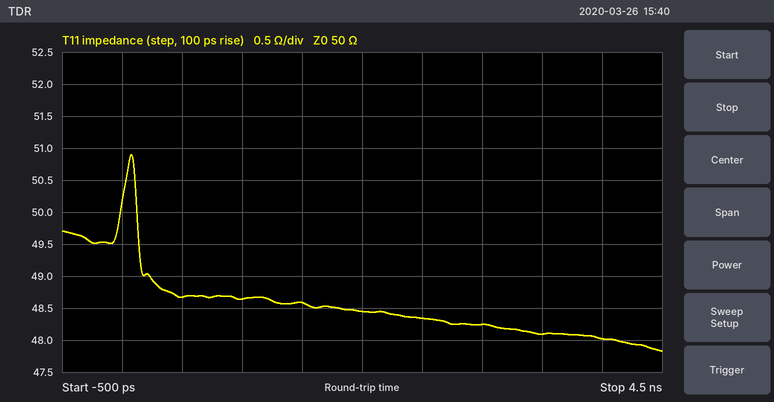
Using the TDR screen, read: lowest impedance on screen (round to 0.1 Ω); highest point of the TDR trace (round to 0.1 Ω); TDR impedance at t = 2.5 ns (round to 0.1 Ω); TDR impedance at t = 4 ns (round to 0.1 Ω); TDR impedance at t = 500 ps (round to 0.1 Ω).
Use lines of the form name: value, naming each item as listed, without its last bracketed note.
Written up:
lowest impedance on screen: 47.8 Ω
highest point of the TDR trace: 50.9 Ω
TDR impedance at t = 2.5 ns: 48.3 Ω
TDR impedance at t = 4 ns: 48.0 Ω
TDR impedance at t = 500 ps: 48.7 Ω
